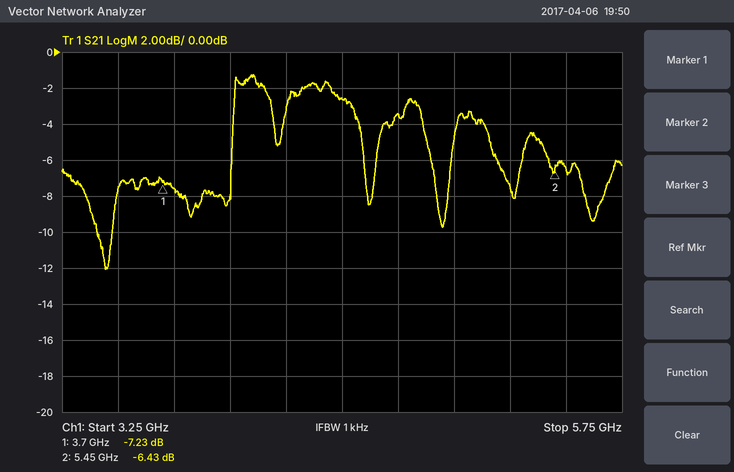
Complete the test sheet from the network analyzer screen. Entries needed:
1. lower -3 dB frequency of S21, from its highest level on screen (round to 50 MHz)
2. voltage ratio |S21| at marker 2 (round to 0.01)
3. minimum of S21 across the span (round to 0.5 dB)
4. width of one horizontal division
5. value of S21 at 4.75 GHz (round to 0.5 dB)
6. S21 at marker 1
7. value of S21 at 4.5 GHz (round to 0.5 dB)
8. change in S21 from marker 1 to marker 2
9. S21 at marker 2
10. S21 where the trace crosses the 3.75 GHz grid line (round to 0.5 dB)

4.00 GHz
0.48
-12.0 dB
250 MHz
-3.5 dB
-7.23 dB
-2.5 dB
0.80 dB
-6.43 dB
-7.5 dB
